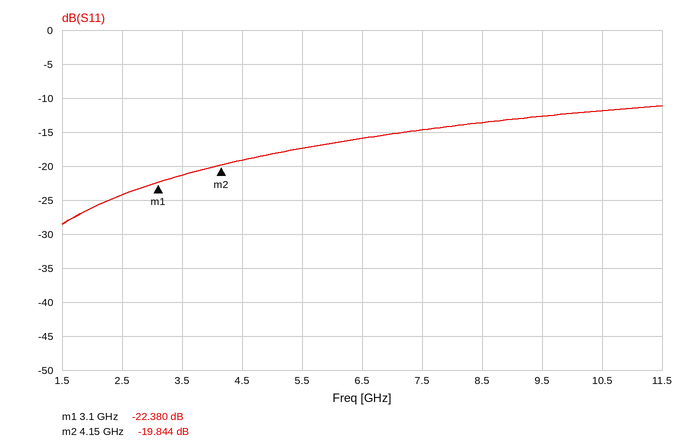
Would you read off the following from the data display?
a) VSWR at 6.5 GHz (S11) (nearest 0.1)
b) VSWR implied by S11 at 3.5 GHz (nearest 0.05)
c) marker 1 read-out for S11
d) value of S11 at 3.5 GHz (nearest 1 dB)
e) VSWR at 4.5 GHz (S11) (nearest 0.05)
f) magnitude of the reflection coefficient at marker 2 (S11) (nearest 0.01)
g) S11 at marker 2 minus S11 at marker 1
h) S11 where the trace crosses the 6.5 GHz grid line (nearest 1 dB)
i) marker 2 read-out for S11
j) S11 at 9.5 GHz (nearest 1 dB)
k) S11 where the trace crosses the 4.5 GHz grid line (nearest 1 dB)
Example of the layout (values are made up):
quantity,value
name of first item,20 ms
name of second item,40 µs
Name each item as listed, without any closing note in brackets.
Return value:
quantity,value
VSWR at 6.5 GHz (S11),1.4
VSWR implied by S11 at 3.5 GHz,1.20
marker 1 read-out for S11,-22.380 dB
value of S11 at 3.5 GHz,-21 dB
VSWR at 4.5 GHz (S11),1.25
magnitude of the reflection coefficient at marker 2 (S11),0.10
S11 at marker 2 minus S11 at marker 1,2.536 dB
S11 where the trace crosses the 6.5 GHz grid line,-16 dB
marker 2 read-out for S11,-19.844 dB
S11 at 9.5 GHz,-13 dB
S11 where the trace crosses the 4.5 GHz grid line,-19 dB
